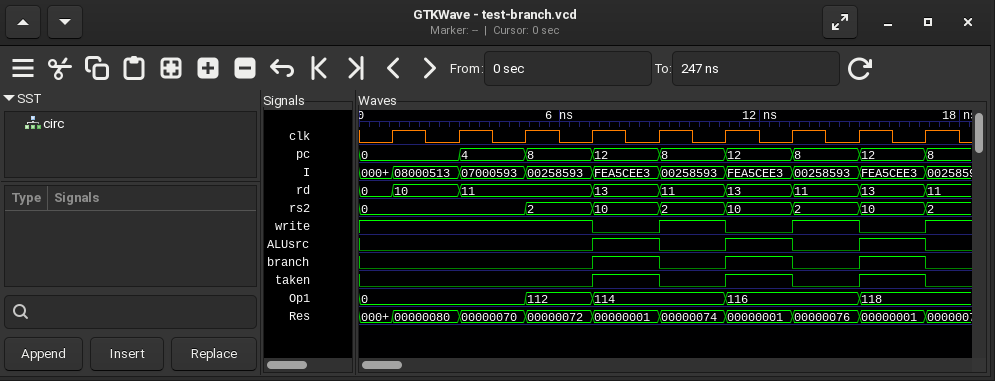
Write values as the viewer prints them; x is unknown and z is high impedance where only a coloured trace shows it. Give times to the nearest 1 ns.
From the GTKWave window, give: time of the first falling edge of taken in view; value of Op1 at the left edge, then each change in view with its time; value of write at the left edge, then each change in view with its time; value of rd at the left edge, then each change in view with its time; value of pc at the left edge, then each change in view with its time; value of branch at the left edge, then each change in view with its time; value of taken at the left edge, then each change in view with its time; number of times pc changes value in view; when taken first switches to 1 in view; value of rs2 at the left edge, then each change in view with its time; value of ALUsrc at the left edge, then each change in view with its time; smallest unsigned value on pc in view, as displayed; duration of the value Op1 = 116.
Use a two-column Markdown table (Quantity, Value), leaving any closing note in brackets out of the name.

| Quantity | Value |
|---|---|
| time of the first falling edge of taken in view | 9 ns |
| value of Op1 at the left edge, then each change in view with its time | 0, 112 at 5 ns, 114 at 7 ns, 116 at 11 ns, 118 at 15 ns |
| value of write at the left edge, then each change in view with its time | 1, 0 at 7 ns, 1 at 9 ns, 0 at 11 ns, 1 at 13 ns, 0 at 15 ns, 1 at 17 ns |
| value of rd at the left edge, then each change in view with its time | 0, 10 at 1 ns, 11 at 3 ns, 13 at 7 ns, 11 at 9 ns, 13 at 11 ns, 11 at 13 ns, 13 at 15 ns, 11 at 17 ns |
| value of pc at the left edge, then each change in view with its time | 0, 4 at 3 ns, 8 at 5 ns, 12 at 7 ns, 8 at 9 ns, 12 at 11 ns, 8 at 13 ns, 12 at 15 ns, 8 at 17 ns |
| value of branch at the left edge, then each change in view with its time | 0, 1 at 7 ns, 0 at 9 ns, 1 at 11 ns, 0 at 13 ns, 1 at 15 ns, 0 at 17 ns |
| value of taken at the left edge, then each change in view with its time | 0, 1 at 7 ns, 0 at 9 ns, 1 at 11 ns, 0 at 13 ns, 1 at 15 ns, 0 at 17 ns |
| number of times pc changes value in view | 8 |
| when taken first switches to 1 in view | 7 ns |
| value of rs2 at the left edge, then each change in view with its time | 0, 2 at 5 ns, 10 at 7 ns, 2 at 9 ns, 10 at 11 ns, 2 at 13 ns, 10 at 15 ns, 2 at 17 ns |
| value of ALUsrc at the left edge, then each change in view with its time | 0, 1 at 7 ns, 0 at 9 ns, 1 at 11 ns, 0 at 13 ns, 1 at 15 ns, 0 at 17 ns |
| smallest unsigned value on pc in view, as displayed | 0 |
| duration of the value Op1 = 116 | 4 ns |
